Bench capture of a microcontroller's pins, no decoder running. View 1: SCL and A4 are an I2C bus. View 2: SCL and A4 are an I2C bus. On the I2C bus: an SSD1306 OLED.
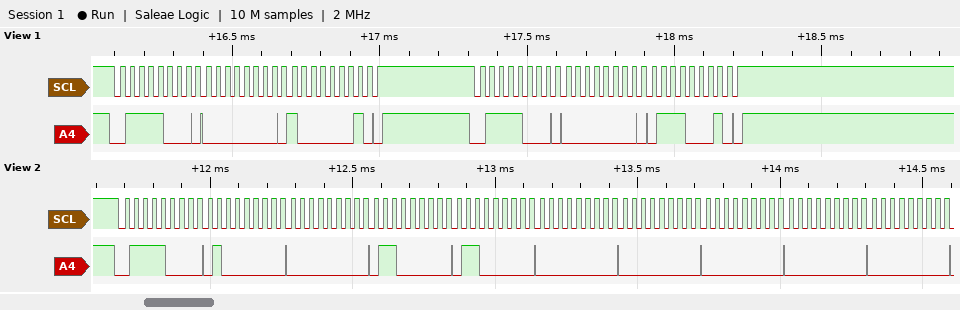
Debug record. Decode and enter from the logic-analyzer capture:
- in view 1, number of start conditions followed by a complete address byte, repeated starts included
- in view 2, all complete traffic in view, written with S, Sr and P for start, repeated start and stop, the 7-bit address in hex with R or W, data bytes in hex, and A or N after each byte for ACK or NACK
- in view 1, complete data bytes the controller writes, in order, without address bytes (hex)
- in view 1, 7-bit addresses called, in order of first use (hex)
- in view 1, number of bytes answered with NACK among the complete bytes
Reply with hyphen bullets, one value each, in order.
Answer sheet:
- 2
- S 3CW A 40 A 00 A 60 A 60 A 00 A 00 A 00 A 00 A 00 A
- 00 81 00 71
- 0x3C
- 0
